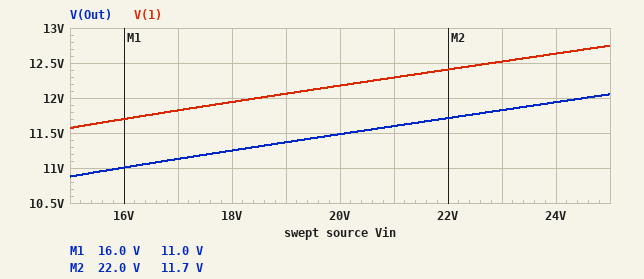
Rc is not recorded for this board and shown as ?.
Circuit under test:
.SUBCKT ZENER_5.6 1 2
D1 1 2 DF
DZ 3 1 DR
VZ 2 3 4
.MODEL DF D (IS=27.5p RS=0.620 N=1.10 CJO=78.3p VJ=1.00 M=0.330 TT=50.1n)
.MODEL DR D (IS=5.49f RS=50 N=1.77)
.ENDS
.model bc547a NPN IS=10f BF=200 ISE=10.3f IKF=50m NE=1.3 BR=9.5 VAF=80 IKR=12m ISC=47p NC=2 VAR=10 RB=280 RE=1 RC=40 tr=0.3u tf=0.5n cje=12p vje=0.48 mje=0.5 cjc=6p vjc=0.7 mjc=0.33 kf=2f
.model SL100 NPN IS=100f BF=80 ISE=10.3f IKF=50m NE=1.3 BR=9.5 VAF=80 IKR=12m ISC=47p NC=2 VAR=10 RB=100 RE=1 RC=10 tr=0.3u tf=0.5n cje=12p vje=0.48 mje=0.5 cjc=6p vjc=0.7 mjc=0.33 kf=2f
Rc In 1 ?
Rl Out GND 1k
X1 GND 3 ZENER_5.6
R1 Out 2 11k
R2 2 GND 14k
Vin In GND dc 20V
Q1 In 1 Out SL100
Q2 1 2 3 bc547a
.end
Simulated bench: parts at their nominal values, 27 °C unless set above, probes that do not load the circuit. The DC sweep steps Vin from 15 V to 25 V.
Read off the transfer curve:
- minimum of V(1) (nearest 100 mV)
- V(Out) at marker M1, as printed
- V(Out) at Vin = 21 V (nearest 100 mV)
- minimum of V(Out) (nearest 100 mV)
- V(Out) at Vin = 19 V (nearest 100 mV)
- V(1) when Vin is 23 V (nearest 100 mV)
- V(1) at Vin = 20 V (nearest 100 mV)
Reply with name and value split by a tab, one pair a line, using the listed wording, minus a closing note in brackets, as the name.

minimum of V(1)	11.6 V
V(Out) at marker M1, as printed	11.0 V
V(Out) at Vin = 21 V	11.6 V
minimum of V(Out)	10.9 V
V(Out) at Vin = 19 V	11.4 V
V(1) when Vin is 23 V	12.5 V
V(1) at Vin = 20 V	12.2 V
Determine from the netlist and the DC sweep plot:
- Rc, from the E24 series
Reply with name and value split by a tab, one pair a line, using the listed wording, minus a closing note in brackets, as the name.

Rc, from the E24 series	1.6 kΩ
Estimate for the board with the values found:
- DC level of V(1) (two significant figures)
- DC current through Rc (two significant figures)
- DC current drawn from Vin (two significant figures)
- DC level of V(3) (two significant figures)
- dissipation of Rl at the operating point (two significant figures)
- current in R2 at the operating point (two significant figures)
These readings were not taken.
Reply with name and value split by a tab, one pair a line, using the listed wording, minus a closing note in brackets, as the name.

DC level of V(1)	12 V
DC current through Rc	4.9 mA
DC current drawn from Vin	17 mA
DC level of V(3)	5.5 V
dissipation of Rl at the operating point	130 mW
current in R2 at the operating point	440 µA
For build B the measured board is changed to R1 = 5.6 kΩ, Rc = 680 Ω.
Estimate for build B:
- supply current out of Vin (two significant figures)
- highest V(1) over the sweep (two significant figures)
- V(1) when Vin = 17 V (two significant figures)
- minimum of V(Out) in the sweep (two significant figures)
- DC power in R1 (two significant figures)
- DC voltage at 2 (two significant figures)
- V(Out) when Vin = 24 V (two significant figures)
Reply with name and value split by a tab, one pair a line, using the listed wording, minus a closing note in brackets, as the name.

supply current out of Vin	24 mA
highest V(1) over the sweep	12 V
V(1) when Vin = 17 V	10 V
minimum of V(Out) in the sweep	9.3 V
DC power in R1	2.0 mW
DC voltage at 2	6.8 V
V(Out) when Vin = 24 V	11 V
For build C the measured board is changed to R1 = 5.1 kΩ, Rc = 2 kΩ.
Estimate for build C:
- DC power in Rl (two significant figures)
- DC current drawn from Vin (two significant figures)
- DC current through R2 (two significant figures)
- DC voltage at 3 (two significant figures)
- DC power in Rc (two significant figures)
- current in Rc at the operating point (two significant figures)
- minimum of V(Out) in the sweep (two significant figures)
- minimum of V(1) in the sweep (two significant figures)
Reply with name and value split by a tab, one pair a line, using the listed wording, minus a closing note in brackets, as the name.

DC power in Rl	76 mW
DC current drawn from Vin	14 mA
DC current through R2	450 µA
DC voltage at 3	5.5 V
DC power in Rc	56 mW
current in Rc at the operating point	5.3 mA
minimum of V(Out) in the sweep	8.4 V
minimum of V(1) in the sweep	9.1 V
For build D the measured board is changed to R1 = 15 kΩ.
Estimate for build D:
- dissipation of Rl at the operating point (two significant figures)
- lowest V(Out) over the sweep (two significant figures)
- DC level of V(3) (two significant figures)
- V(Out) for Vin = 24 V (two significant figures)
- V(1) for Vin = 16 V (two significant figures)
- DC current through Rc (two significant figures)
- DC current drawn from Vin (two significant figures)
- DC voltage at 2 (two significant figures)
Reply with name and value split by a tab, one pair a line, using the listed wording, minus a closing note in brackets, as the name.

dissipation of Rl at the operating point	170 mW
lowest V(Out) over the sweep	12 V
DC level of V(3)	5.4 V
V(Out) for Vin = 24 V	14 V
V(1) for Vin = 16 V	13 V
DC current through Rc	3.9 mA
DC current drawn from Vin	17 mA
DC voltage at 2	6.1 V
